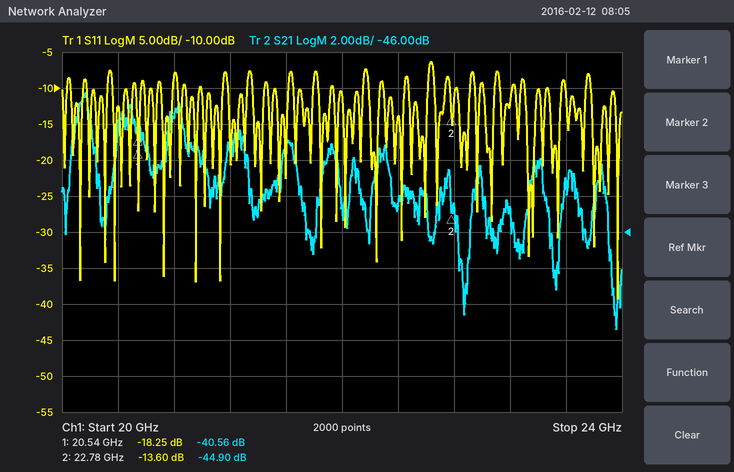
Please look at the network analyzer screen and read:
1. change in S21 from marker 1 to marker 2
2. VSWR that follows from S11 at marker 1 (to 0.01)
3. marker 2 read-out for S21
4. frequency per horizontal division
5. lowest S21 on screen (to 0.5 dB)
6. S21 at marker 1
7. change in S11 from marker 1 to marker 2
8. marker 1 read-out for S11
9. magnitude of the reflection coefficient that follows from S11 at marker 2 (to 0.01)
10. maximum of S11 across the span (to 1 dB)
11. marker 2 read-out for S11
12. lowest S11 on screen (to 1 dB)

-4.34 dB
1.28
-44.90 dB
400 MHz
-51.5 dB
-40.56 dB
4.65 dB
-18.25 dB
0.21
-6 dB
-13.60 dB
-39 dB
